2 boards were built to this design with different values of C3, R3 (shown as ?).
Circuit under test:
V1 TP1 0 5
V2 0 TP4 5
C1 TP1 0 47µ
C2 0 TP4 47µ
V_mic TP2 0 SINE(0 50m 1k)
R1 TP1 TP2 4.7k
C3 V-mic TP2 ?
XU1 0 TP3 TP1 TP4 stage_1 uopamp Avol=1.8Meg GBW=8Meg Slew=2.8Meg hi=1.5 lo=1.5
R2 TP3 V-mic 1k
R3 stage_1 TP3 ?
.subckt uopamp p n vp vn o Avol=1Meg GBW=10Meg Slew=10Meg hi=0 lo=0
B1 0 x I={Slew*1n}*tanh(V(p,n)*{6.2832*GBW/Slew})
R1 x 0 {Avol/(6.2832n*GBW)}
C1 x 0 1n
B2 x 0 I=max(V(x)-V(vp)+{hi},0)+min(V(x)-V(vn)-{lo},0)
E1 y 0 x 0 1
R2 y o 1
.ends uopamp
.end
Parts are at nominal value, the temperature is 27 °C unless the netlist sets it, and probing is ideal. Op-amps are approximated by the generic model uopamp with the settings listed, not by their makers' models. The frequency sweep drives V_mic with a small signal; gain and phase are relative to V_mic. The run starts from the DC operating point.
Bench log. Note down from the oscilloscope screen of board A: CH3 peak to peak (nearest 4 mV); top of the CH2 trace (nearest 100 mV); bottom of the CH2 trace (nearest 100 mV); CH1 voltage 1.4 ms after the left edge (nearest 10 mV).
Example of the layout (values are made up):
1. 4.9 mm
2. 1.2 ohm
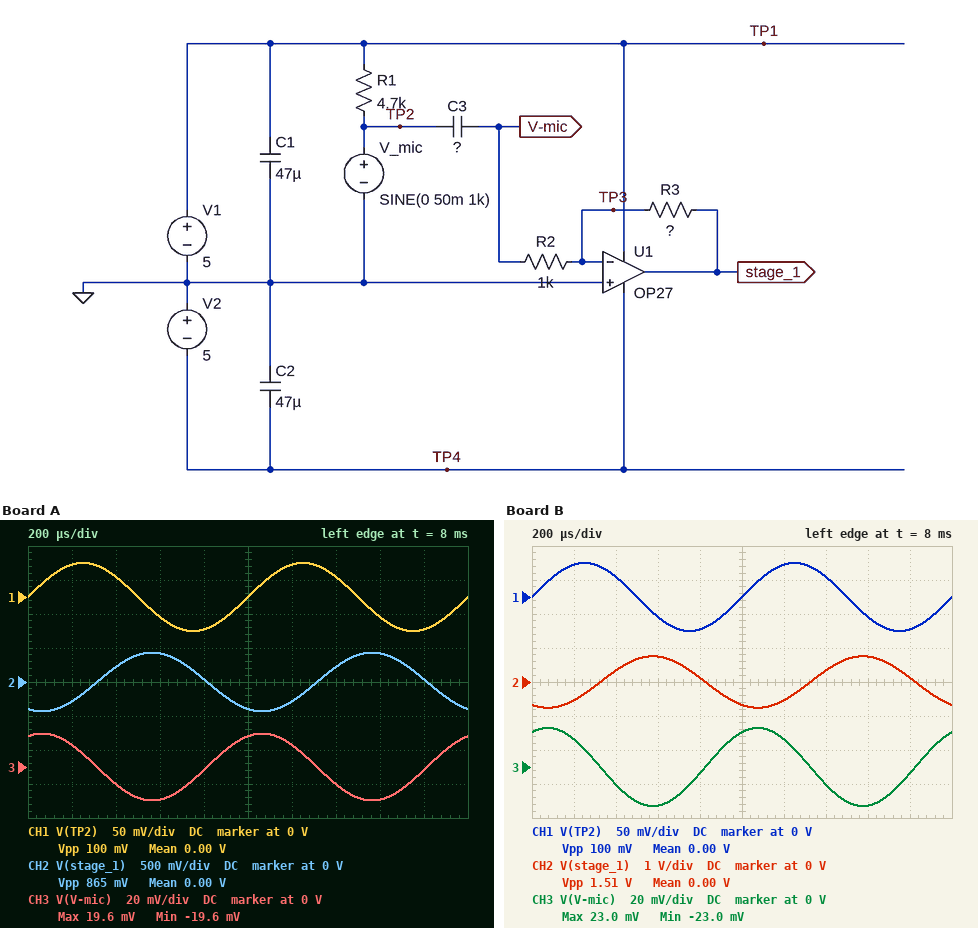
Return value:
1. 40 mV
2. 400 mV
3. -400 mV
4. 30 mV
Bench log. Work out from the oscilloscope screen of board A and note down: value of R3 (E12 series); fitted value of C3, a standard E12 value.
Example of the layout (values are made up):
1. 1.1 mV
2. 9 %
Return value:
1. 22 kΩ
2. 68 nF
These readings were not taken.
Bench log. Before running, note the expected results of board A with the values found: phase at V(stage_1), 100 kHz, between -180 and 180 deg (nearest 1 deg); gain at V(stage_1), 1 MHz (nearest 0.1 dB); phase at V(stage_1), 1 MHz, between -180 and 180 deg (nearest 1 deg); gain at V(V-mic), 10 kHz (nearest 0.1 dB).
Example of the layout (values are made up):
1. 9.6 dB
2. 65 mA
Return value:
1. 165 deg
2. 17.2 dB
3. 109 deg
4. -0.2 dB
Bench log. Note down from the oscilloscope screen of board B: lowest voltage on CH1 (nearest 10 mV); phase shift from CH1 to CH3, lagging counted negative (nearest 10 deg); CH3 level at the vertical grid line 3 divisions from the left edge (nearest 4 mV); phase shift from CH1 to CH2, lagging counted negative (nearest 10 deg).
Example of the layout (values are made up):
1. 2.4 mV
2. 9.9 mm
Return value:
1. -50 mV
2. 60 deg
3. -24 mV
4. -120 deg
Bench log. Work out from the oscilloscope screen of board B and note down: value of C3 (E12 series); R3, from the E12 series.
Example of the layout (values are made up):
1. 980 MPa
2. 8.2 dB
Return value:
1. 82 nF
2. 33 kΩ
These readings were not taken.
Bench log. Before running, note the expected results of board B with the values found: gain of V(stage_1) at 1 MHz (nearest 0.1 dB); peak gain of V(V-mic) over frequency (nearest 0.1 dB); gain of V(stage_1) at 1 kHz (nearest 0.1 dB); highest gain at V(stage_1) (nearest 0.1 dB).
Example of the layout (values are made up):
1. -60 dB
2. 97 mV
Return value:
1. 17.6 dB
2. 0.1 dB
3. 23.6 dB
4. 30.4 dB
